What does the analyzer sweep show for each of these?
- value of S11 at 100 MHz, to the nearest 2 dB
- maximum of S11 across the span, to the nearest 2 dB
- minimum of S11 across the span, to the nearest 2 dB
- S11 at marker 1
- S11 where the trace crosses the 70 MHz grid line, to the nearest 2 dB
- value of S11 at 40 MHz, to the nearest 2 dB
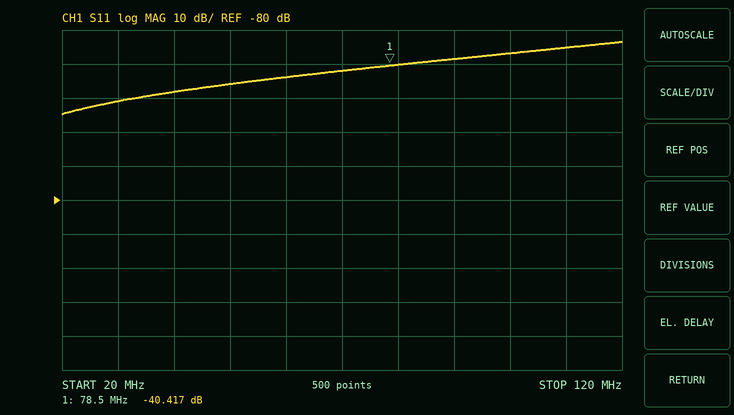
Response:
-36 dB
-34 dB
-54 dB
-40.417 dB
-42 dB
-48 dB
